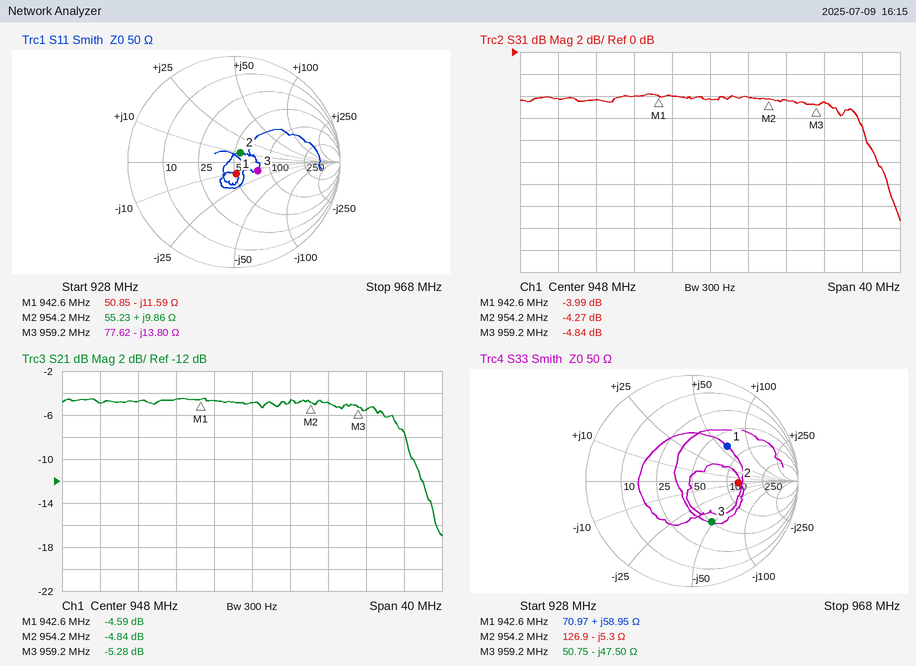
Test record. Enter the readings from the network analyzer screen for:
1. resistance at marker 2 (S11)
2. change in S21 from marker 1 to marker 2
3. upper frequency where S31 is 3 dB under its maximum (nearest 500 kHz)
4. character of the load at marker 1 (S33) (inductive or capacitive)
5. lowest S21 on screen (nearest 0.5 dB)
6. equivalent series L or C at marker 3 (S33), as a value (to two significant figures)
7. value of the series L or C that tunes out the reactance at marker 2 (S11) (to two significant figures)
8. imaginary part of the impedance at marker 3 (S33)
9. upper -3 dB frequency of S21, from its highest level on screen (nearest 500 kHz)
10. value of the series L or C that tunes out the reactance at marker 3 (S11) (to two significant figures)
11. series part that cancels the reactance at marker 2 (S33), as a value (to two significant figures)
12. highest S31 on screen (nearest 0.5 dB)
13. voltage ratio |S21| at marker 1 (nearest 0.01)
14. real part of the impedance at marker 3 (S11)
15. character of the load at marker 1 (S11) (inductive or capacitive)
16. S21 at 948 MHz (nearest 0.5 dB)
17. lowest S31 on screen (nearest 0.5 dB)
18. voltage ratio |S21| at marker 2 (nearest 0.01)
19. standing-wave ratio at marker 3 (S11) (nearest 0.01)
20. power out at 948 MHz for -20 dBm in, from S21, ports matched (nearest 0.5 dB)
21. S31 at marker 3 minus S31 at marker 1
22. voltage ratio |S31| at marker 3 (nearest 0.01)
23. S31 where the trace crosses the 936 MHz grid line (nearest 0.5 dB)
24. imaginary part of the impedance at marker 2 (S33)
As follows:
55.23 Ω
-0.25 dB
964.0 MHz
inductive
-17.0 dB
3.5 pF
17 pF
-47.50 Ω
964.0 MHz
2.3 nH
880 pH
-4.0 dB
0.59
77.62 Ω
capacitive
-5.0 dB
-15.5 dB
0.57
1.63
-25.0 dBm
-0.85 dB
0.57
-4.5 dB
-5.3 Ω
